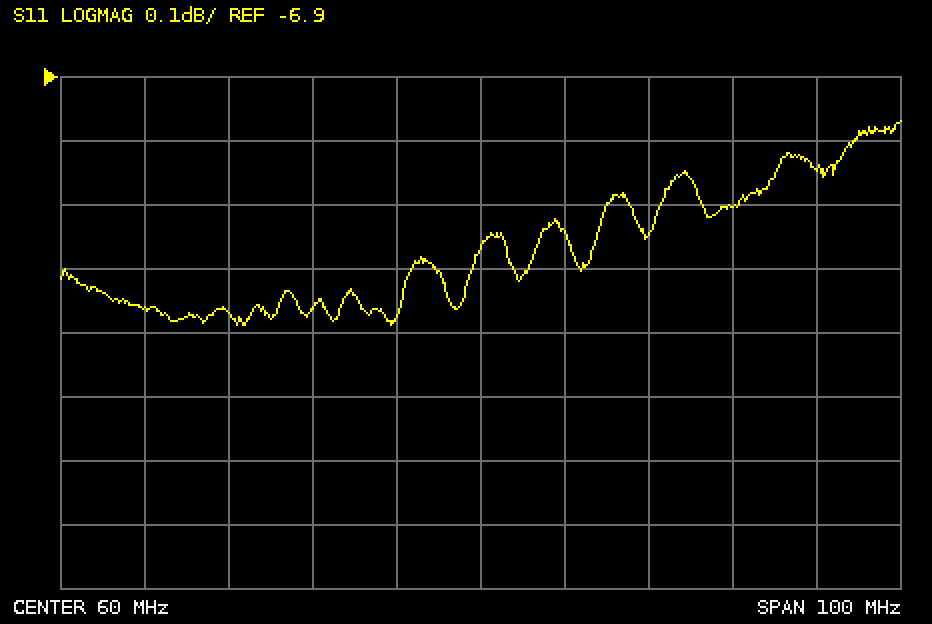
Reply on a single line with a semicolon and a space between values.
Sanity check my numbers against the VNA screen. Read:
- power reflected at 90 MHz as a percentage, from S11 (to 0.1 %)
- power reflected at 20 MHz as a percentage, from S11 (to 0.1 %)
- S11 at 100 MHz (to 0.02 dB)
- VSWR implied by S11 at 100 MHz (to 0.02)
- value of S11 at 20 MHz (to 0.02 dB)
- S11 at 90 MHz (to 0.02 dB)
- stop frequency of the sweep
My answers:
19.5 %; 18.8 %; -7.04 dB; 2.60; -7.26 dB; -7.10 dB; 110 MHz
